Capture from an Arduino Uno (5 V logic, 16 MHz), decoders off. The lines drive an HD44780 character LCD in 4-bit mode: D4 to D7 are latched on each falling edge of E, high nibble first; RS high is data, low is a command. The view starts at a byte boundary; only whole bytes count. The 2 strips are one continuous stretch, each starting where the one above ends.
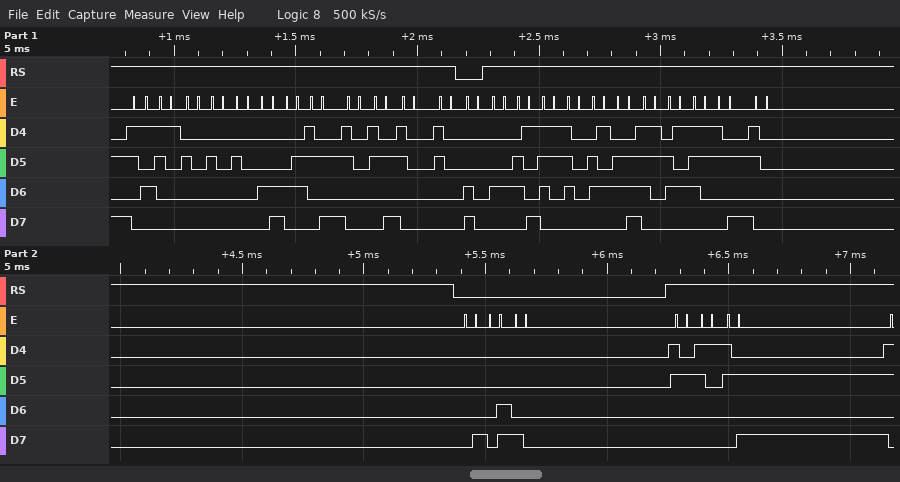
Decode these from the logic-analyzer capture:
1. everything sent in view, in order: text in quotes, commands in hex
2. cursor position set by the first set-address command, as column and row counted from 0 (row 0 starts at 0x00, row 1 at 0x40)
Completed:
"51   LF:0:00" 0xC0 "Dispenses:0" 0x08 0x0C 0x80 "21:"
column 0, row 1
